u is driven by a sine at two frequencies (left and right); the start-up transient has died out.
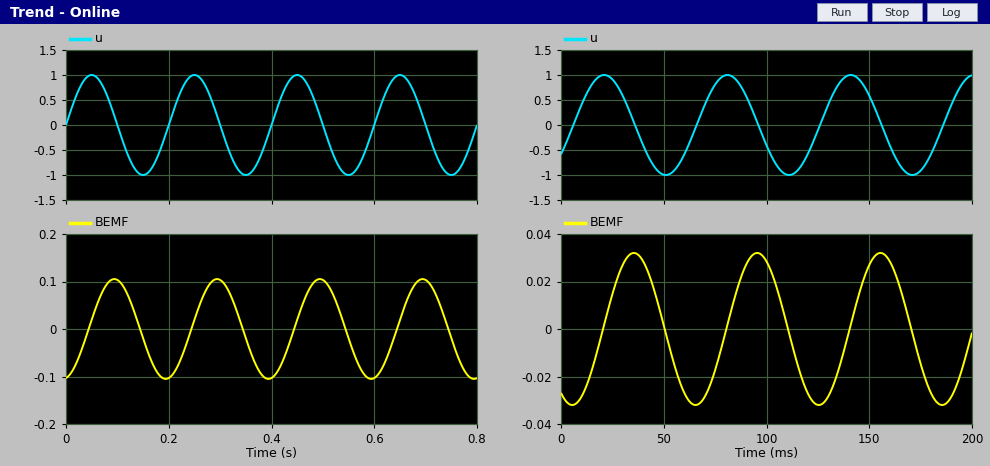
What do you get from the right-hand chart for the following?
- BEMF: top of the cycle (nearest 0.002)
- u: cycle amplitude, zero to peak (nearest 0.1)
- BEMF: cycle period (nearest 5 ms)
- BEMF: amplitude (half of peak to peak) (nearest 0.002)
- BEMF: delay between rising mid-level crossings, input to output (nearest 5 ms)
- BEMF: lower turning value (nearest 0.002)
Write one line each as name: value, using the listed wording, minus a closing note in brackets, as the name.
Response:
BEMF: top of the cycle: 0.032
u: cycle amplitude, zero to peak: 1.0
BEMF: cycle period: 60 ms
BEMF: amplitude (half of peak to peak): 0.032
BEMF: delay between rising mid-level crossings, input to output: 15 ms
BEMF: lower turning value: -0.032
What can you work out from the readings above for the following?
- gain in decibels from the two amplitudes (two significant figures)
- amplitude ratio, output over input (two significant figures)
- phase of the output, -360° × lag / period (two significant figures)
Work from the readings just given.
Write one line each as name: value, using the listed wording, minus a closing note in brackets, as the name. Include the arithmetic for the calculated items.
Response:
gain in decibels from the two amplitudes: 20 log10(0.032 / 1) = -30 dB
amplitude ratio, output over input: 0.032 / 1 = 0.032
phase of the output, -360° × lag / period: -360 × 15 / 60 = -90°
